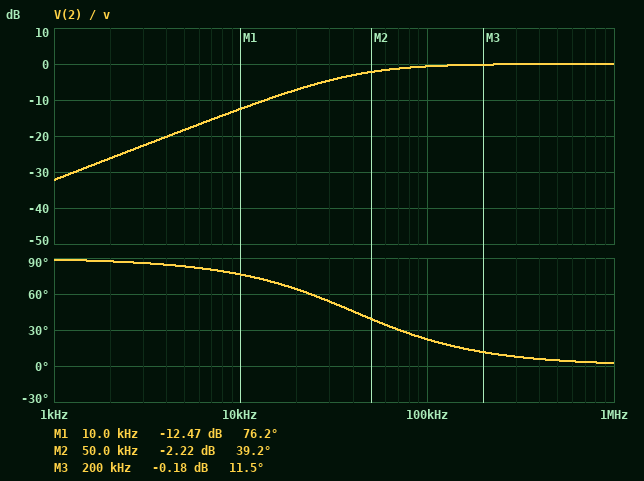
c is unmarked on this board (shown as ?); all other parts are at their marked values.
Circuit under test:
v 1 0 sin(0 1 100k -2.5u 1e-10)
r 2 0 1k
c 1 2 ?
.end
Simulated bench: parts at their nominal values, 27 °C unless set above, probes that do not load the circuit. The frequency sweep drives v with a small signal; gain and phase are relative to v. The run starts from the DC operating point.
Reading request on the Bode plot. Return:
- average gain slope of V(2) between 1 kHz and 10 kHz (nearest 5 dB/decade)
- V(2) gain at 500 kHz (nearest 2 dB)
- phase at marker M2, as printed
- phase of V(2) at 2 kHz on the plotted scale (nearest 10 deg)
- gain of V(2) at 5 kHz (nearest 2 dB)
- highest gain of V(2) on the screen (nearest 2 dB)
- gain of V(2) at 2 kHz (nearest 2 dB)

20 dB/decade
0 dB
39.2 deg
90 deg
-18 dB
0 dB
-26 dB
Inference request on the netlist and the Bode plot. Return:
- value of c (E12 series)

3.9 nF
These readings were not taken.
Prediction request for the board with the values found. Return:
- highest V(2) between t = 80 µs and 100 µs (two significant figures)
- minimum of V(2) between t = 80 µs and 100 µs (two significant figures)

930 mV
-930 mV
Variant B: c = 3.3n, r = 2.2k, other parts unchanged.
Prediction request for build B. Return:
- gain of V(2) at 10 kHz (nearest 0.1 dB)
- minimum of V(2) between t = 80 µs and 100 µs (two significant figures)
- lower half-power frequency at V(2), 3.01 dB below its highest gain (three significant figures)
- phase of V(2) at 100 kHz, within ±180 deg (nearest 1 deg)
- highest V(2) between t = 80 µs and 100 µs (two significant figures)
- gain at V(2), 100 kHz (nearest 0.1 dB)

-7.6 dB
-980 mV
21.9 kHz
12 deg
980 mV
-0.2 dB
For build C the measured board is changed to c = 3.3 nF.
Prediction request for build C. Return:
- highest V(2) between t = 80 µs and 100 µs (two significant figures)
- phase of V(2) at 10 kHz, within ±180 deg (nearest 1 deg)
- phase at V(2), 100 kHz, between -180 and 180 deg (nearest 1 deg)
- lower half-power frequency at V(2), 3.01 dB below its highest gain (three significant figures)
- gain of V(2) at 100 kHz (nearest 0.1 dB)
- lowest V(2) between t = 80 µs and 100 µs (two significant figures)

900 mV
78 deg
26 deg
48.2 kHz
-0.9 dB
-900 mV
